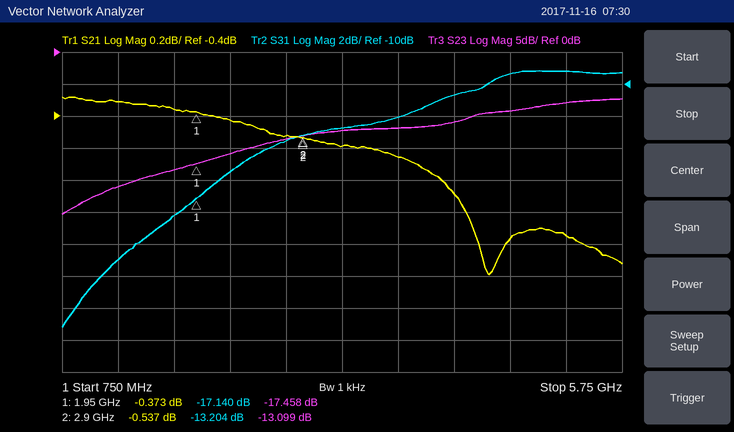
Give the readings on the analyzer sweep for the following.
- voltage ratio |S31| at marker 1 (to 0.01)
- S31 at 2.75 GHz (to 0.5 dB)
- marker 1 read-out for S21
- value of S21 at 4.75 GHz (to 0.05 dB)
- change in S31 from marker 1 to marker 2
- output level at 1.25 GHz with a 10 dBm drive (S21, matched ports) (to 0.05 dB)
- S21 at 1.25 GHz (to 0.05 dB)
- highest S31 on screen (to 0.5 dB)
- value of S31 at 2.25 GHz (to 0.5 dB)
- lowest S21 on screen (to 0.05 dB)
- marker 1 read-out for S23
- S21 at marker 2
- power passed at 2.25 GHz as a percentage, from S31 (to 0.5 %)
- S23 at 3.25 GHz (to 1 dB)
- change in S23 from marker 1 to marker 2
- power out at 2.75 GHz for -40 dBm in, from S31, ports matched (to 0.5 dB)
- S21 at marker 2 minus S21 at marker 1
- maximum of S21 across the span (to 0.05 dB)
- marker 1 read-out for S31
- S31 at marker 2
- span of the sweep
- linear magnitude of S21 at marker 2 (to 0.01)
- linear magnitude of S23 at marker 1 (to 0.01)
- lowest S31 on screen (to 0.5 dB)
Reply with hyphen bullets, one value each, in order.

- 0.14
- -13.5 dB
- -0.373 dB
- -1.15 dB
- 3.936 dB
- 9.70 dBm
- -0.30 dB
- -9.0 dB
- -15.5 dB
- -1.40 dB
- -17.458 dB
- -0.537 dB
- 3.0 %
- -12 dB
- 4.359 dB
- -53.5 dBm
- -0.164 dB
- -0.30 dB
- -17.140 dB
- -13.204 dB
- 5 GHz
- 0.94
- 0.13
- -25.0 dB
